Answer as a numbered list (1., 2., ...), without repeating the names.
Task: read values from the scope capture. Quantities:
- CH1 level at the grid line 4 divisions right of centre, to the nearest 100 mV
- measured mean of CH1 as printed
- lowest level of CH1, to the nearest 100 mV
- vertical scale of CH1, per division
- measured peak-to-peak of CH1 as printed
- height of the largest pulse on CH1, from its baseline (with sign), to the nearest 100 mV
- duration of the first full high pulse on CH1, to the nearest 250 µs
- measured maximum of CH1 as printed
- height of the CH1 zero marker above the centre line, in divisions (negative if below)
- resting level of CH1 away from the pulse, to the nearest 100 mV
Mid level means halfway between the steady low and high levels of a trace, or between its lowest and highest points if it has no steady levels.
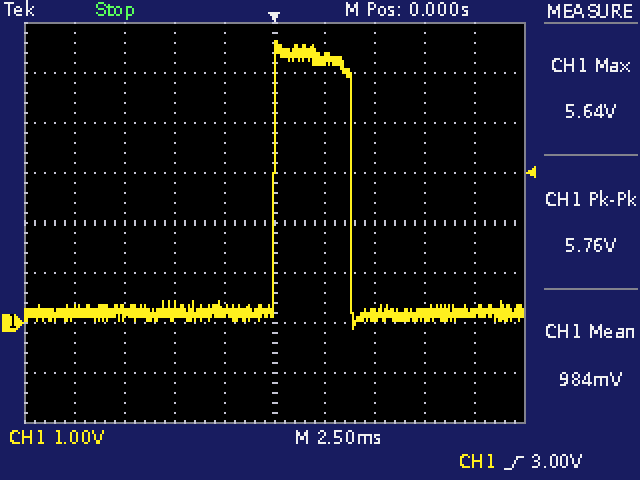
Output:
1. 200 mV
2. 984 mV
3. -100 mV
4. 1 V
5. 5.76 V
6. +5.4 V
7. 3.75 ms
8. 5.64 V
9. -2.0 div
10. 200 mV
